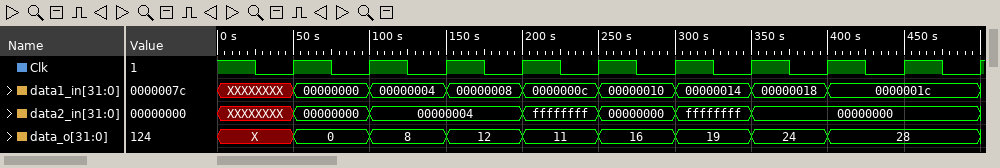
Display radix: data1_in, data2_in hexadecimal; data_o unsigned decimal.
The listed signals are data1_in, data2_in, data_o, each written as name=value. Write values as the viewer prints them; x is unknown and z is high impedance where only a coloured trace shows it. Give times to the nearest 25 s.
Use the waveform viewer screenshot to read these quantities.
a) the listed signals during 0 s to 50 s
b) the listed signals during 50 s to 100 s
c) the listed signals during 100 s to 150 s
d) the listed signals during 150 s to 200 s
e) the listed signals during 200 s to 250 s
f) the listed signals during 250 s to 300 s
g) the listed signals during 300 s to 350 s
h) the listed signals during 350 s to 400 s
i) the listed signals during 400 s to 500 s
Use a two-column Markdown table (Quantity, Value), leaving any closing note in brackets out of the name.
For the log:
| Quantity | Value |
|---|---|
| the listed signals during 0 s to 50 s | data1_in=XXXXXXXX, data2_in=XXXXXXXX, data_o=X |
| the listed signals during 50 s to 100 s | data1_in=00000000, data2_in=00000000, data_o=0 |
| the listed signals during 100 s to 150 s | data1_in=00000004, data2_in=00000004, data_o=8 |
| the listed signals during 150 s to 200 s | data1_in=00000008, data2_in=00000004, data_o=12 |
| the listed signals during 200 s to 250 s | data1_in=0000000c, data2_in=ffffffff, data_o=11 |
| the listed signals during 250 s to 300 s | data1_in=00000010, data2_in=00000000, data_o=16 |
| the listed signals during 300 s to 350 s | data1_in=00000014, data2_in=ffffffff, data_o=19 |
| the listed signals during 350 s to 400 s | data1_in=00000018, data2_in=00000000, data_o=24 |
| the listed signals during 400 s to 500 s | data1_in=0000001c, data2_in=00000000, data_o=28 |
